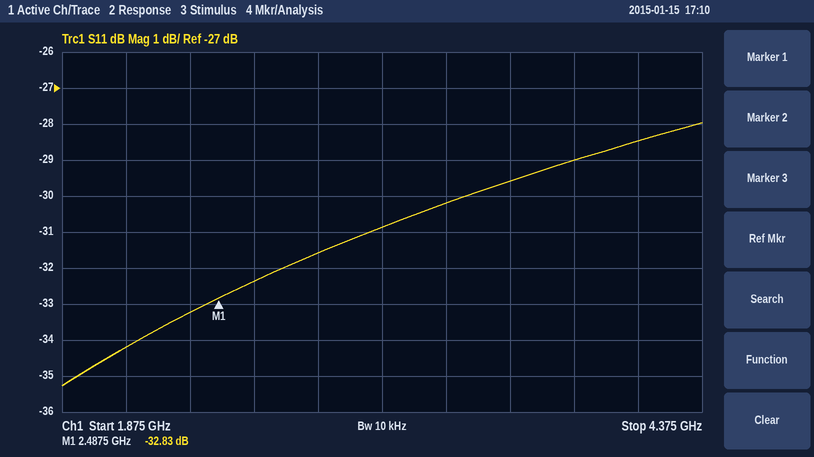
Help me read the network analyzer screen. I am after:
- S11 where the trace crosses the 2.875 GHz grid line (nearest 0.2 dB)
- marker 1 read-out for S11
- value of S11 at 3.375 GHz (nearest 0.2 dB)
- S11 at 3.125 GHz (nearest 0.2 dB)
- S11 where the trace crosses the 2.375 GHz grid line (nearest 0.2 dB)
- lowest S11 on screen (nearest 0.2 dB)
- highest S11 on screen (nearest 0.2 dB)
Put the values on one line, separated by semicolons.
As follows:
-31.6 dB; -32.83 dB; -30.2 dB; -30.8 dB; -33.2 dB; -35.2 dB; -28.0 dB
